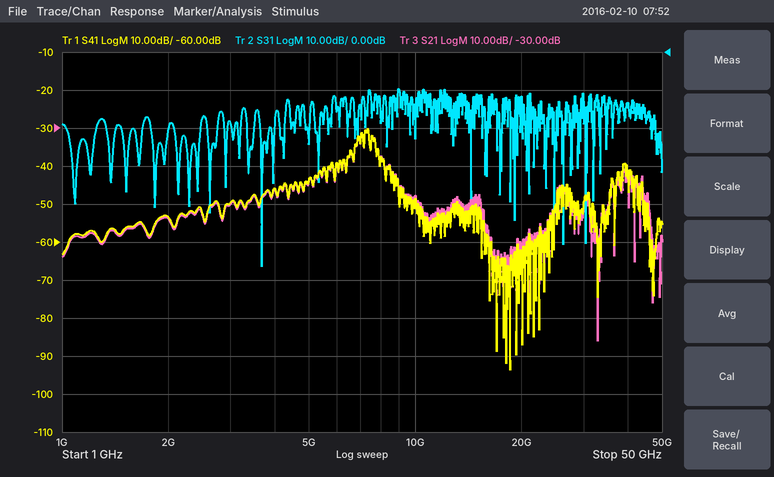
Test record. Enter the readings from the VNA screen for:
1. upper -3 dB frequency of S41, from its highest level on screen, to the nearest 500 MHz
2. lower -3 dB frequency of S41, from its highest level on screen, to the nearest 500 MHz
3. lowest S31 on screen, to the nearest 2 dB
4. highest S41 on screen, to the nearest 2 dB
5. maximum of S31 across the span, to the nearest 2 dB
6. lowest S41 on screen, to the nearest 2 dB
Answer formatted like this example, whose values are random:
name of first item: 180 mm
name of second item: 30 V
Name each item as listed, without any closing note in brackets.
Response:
upper -3 dB frequency of S41, from its highest level on screen, to the nearest 500 MHz: 7.5 GHz
lower -3 dB frequency of S41, from its highest level on screen, to the nearest 500 MHz: 7.0 GHz
lowest S31 on screen, to the nearest 2 dB: -56 dB
highest S41 on screen, to the nearest 2 dB: -30 dB
maximum of S31 across the span, to the nearest 2 dB: -10 dB
lowest S41 on screen, to the nearest 2 dB: -94 dB
